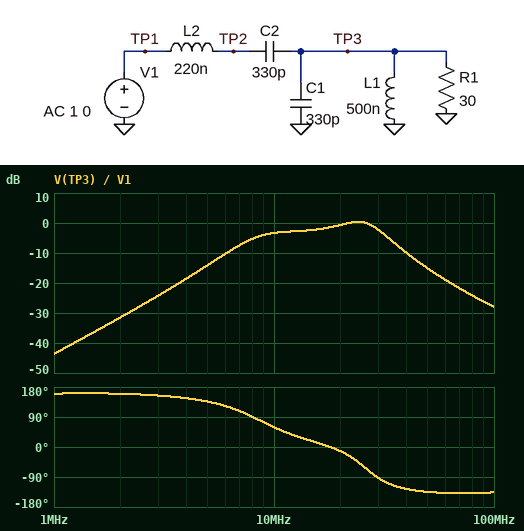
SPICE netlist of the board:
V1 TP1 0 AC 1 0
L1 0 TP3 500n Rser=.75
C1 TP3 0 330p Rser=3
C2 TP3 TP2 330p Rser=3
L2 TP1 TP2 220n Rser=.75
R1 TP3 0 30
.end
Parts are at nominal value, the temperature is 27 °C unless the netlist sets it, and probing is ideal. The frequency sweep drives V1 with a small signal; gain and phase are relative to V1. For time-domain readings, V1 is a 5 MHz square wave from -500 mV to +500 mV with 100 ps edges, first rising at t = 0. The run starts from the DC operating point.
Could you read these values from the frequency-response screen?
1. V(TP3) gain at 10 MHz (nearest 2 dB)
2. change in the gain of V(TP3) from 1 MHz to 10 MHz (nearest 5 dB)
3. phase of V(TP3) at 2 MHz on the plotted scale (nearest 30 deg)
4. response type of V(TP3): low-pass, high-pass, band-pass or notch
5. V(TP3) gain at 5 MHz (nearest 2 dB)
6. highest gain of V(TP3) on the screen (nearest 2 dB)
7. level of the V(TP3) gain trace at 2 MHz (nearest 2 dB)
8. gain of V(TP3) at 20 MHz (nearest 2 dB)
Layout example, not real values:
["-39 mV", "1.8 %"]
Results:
["-4 dB", "40 dB", "150 deg", "band-pass", "-14 dB", "0 dB", "-32 dB", "0 dB"]
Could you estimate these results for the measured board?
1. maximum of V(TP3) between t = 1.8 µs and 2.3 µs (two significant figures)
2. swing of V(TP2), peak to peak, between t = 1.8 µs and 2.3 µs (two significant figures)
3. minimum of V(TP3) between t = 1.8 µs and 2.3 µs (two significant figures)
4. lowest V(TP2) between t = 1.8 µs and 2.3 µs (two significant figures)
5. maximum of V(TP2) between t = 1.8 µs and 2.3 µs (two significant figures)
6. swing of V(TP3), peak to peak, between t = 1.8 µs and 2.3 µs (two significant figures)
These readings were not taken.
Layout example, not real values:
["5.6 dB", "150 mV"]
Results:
["380 mV", "2.0 V", "-380 mV", "-1.0 V", "1.0 V", "770 mV"]
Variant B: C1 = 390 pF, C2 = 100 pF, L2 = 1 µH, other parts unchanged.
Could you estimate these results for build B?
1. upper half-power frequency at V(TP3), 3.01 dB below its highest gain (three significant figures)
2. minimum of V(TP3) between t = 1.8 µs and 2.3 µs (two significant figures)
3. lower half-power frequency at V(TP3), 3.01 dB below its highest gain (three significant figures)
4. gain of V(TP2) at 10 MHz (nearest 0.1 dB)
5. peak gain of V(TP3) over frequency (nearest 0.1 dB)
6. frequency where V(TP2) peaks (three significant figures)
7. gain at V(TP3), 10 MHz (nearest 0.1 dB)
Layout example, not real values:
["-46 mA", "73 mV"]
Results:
["18.8 MHz", "-200 mV", "14.7 MHz", "4.3 dB", "-0.3 dB", "16.9 MHz", "-10.9 dB"]
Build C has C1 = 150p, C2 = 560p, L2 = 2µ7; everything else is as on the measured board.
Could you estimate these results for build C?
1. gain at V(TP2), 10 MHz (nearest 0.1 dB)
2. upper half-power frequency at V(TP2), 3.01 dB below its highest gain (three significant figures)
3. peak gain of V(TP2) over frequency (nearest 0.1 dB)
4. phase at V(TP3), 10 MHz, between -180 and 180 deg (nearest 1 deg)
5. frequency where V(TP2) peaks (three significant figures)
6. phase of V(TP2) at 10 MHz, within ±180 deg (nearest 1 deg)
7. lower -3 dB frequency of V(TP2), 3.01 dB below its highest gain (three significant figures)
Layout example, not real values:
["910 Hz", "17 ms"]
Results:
["-15.0 dB", "3.99 MHz", "17.6 dB", "-48 deg", "3.78 MHz", "-114 deg", "3.54 MHz"]
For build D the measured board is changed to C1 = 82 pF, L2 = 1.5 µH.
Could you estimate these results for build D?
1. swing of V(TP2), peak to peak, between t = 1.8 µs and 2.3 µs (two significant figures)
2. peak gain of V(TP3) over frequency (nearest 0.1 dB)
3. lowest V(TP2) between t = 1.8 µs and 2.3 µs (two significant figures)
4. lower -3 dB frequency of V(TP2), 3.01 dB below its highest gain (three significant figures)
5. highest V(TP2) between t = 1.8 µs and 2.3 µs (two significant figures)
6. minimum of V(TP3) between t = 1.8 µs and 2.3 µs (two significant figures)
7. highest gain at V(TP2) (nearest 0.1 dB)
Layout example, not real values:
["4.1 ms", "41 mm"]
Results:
["2.8 V", "1.7 dB", "-1.4 V", "5.63 MHz", "1.4 V", "-250 mV", "13.0 dB"]
